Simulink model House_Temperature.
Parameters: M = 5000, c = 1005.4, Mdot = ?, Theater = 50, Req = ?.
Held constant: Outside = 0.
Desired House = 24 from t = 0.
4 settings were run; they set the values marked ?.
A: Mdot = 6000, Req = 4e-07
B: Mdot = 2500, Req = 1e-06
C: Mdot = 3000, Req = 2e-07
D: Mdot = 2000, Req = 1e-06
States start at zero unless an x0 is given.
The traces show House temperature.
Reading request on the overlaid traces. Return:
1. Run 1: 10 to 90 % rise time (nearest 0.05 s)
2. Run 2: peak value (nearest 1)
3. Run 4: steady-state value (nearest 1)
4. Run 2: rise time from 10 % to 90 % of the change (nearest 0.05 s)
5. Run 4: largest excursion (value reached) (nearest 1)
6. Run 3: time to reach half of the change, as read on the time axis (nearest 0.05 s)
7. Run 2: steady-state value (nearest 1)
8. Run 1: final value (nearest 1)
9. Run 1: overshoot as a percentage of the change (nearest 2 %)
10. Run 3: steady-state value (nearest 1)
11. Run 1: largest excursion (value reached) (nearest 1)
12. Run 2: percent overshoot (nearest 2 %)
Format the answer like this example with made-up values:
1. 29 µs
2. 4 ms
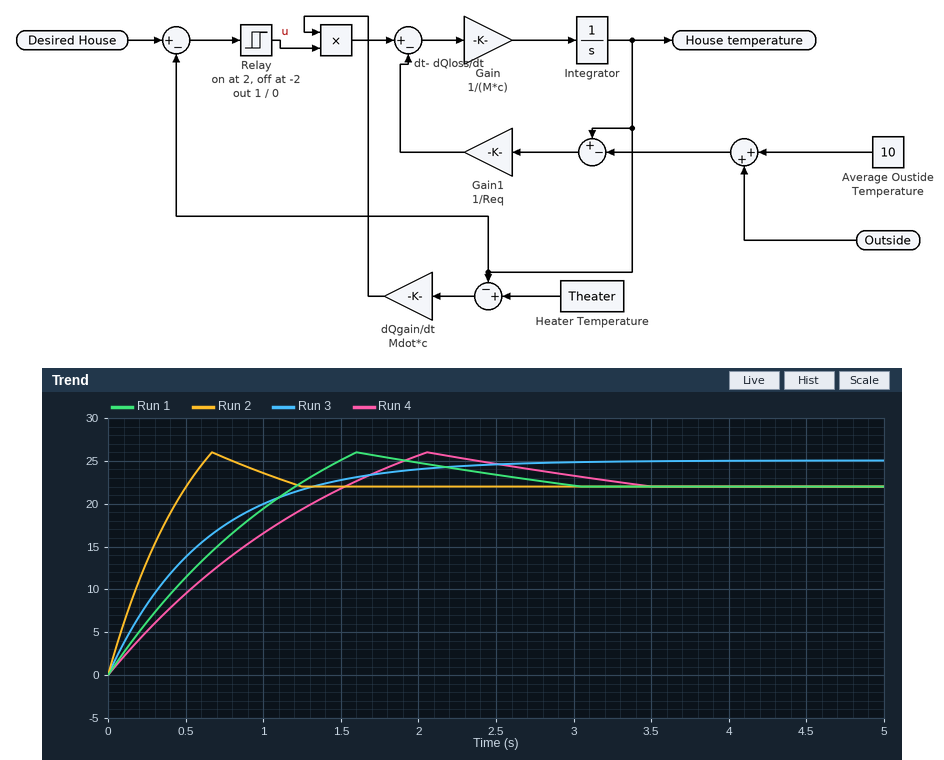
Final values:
1. 0.95 s
2. 26
3. 22
4. 0.40 s
5. 26
6. 0.45 s
7. 22
8. 22
9. 18 %
10. 25
11. 26
12. 18 %
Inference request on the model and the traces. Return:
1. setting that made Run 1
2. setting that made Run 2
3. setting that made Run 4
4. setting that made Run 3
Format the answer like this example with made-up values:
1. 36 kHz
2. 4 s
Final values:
1. B
2. A
3. D
4. C
